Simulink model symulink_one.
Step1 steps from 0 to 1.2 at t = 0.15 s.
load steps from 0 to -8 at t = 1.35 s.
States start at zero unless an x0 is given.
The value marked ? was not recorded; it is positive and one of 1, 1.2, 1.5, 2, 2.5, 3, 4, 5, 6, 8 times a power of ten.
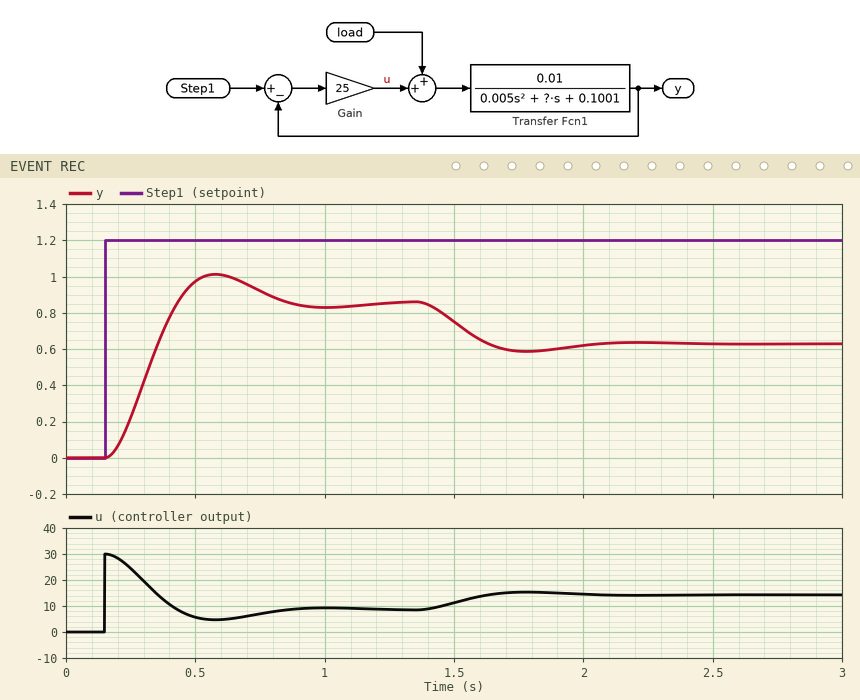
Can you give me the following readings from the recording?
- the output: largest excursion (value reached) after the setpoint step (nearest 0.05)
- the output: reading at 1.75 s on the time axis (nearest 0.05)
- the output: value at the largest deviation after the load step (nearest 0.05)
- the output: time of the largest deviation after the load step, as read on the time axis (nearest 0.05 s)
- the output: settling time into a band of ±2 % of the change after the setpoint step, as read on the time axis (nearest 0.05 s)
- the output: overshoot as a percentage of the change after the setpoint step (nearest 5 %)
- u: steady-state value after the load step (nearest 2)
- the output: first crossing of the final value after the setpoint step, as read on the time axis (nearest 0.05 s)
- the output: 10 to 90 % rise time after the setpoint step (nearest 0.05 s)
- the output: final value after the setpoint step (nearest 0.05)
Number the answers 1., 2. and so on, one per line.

1. 1.00
2. 0.60
3. 0.60
4. 1.80 s
5. 1.15 s
6. 20 %
7. 14
8. 0.45 s
9. 0.20 s
10. 0.85
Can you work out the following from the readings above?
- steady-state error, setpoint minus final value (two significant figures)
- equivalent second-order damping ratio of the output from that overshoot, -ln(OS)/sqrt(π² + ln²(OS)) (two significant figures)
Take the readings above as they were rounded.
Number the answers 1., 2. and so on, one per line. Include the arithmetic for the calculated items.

1. 1.2 - 0.85 = 0.35
2. ln(0.2) = -1.609; 1.609 / sqrt(9.870 + 2.590) = 0.46
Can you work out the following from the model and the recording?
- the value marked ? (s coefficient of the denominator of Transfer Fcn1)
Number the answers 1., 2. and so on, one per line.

1. 0.04
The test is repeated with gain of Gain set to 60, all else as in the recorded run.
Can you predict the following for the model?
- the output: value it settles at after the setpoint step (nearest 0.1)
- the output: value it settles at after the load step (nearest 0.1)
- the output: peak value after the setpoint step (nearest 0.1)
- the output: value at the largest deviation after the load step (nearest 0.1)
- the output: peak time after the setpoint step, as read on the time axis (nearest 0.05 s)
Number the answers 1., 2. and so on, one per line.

1. 1.0
2. 0.9
3. 1.4
4. 0.9
5. 0.45 s
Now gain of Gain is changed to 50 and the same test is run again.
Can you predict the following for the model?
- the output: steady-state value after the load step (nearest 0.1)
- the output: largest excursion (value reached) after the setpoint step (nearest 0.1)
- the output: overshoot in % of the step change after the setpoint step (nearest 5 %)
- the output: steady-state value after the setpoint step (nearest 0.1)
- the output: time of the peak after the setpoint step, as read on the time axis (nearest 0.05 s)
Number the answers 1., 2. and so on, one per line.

1. 0.9
2. 1.3
3. 30 %
4. 1.0
5. 0.45 s
